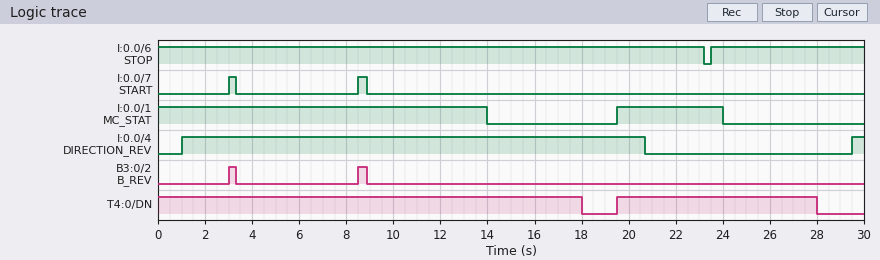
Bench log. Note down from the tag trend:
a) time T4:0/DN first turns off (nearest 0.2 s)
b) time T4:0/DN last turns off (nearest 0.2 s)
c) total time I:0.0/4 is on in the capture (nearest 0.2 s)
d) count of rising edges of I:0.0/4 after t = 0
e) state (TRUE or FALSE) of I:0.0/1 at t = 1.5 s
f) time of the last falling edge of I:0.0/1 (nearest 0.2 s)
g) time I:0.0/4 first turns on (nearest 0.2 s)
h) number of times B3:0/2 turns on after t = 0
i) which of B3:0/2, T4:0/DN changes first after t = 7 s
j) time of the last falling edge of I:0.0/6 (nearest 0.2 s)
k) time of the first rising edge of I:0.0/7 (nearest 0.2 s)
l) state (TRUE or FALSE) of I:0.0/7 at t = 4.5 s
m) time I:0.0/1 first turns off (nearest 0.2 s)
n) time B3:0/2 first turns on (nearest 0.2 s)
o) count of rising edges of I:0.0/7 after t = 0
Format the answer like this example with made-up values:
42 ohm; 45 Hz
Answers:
18.0 s; 28.0 s; 20.2 s; 2; TRUE; 24.0 s; 1.0 s; 2; B3:0/2; 23.2 s; 3.0 s; FALSE; 14.0 s; 3.0 s; 2
